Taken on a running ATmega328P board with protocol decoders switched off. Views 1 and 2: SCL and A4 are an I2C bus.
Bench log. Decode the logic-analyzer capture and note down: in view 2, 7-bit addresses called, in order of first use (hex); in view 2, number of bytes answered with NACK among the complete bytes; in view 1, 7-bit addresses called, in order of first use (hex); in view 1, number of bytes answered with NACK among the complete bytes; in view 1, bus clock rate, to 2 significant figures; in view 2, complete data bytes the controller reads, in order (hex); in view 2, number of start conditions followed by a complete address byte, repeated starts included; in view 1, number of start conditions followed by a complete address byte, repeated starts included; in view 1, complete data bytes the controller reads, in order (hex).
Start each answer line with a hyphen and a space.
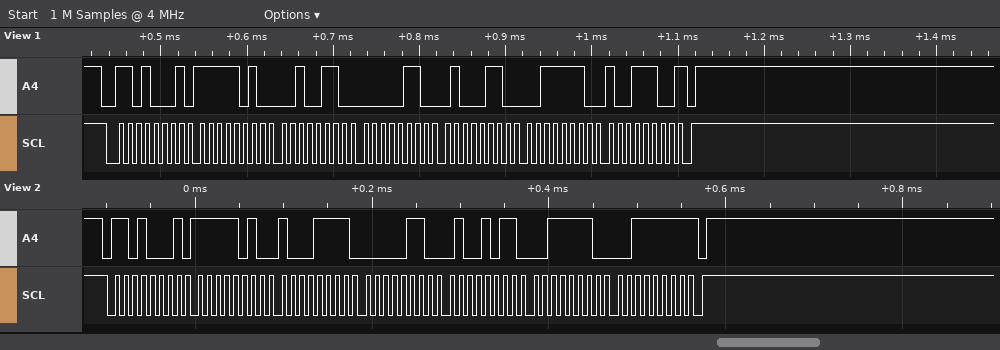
- 0x68
- 1
- 0x68
- 1
- 100 kHz
- FA 8F 06 4B 3E 3F
- 1
- 1
- FA 26 06 46 3E 9C
